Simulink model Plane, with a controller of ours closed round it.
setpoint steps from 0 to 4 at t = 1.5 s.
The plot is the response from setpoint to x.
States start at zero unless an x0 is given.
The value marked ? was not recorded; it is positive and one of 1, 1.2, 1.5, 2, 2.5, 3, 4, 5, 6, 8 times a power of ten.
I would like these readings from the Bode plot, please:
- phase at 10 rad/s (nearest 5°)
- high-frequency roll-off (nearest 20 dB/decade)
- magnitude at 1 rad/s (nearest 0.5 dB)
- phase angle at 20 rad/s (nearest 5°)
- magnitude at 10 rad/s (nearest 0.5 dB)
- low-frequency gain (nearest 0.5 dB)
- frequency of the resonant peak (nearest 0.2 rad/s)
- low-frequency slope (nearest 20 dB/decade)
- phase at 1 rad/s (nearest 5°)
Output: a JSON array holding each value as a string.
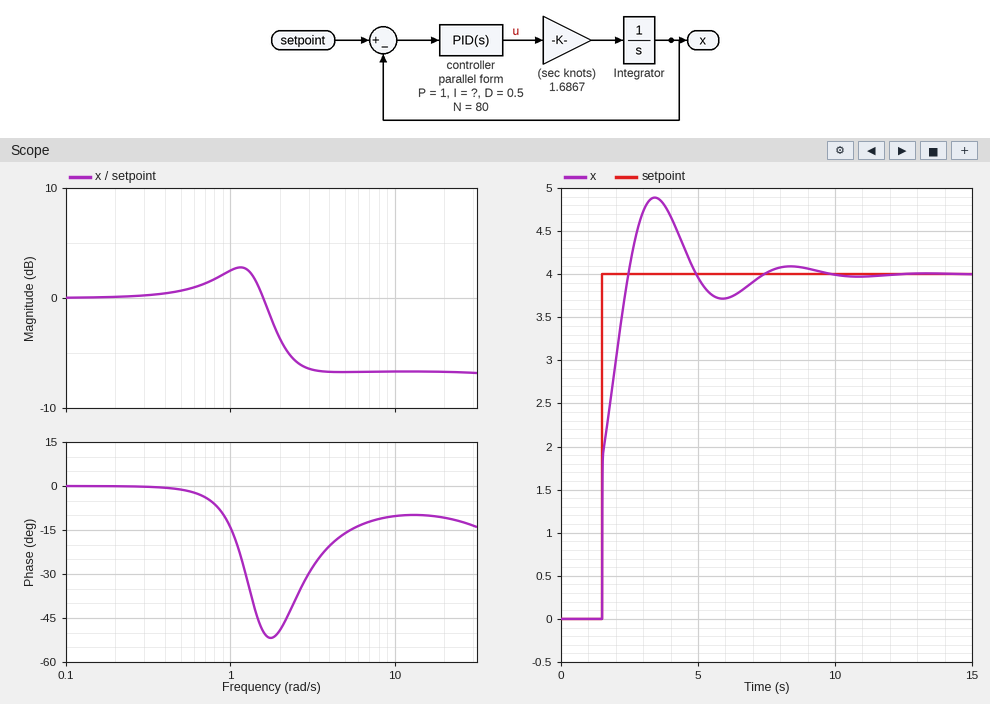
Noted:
["-10°", "0 dB/decade", "2.5 dB", "-10°", "-6.5 dB", "0.0 dB", "1.2 rad/s", "0 dB/decade", "-15°"]
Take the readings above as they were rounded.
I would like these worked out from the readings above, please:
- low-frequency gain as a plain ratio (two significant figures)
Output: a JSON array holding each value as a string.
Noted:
["1.0"]
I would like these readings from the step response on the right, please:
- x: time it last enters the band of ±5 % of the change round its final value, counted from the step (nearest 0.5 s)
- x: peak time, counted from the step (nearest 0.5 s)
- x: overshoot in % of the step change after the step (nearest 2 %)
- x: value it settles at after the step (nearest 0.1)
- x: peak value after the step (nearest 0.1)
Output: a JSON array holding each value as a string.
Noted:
["5.0 s", "2.0 s", "22 %", "4.0", "4.9"]
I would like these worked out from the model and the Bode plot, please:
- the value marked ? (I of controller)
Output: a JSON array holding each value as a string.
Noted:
["2"]
